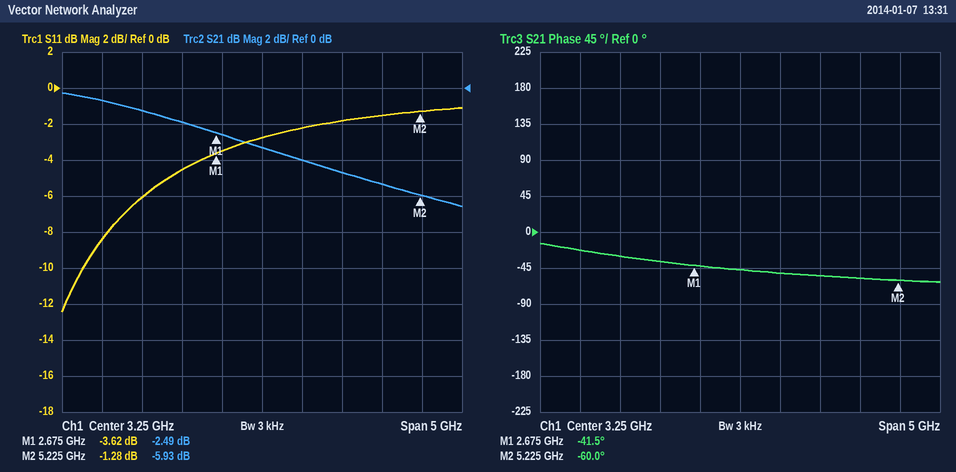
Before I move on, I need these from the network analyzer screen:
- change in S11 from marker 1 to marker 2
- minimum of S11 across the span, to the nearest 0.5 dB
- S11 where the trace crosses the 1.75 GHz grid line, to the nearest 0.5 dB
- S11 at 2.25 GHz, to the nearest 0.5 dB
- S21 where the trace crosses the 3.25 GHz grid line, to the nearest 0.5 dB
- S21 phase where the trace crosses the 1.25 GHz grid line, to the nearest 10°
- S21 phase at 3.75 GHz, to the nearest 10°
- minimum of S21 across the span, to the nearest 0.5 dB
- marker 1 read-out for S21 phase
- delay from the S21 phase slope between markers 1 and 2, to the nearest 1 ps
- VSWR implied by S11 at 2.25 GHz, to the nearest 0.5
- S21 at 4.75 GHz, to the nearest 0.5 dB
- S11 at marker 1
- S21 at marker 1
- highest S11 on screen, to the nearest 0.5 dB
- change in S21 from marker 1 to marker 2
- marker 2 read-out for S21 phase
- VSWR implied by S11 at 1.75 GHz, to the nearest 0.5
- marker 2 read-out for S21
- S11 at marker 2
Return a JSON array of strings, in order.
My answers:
["2.34 dB", "-12.5 dB", "-6.0 dB", "-4.5 dB", "-3.5 dB", "-20°", "-50°", "-6.5 dB", "-41.5°", "20 ps", "4.0", "-5.5 dB", "-3.62 dB", "-2.49 dB", "-1.0 dB", "-3.44 dB", "-60.0°", "3.0", "-5.93 dB", "-1.28 dB"]
